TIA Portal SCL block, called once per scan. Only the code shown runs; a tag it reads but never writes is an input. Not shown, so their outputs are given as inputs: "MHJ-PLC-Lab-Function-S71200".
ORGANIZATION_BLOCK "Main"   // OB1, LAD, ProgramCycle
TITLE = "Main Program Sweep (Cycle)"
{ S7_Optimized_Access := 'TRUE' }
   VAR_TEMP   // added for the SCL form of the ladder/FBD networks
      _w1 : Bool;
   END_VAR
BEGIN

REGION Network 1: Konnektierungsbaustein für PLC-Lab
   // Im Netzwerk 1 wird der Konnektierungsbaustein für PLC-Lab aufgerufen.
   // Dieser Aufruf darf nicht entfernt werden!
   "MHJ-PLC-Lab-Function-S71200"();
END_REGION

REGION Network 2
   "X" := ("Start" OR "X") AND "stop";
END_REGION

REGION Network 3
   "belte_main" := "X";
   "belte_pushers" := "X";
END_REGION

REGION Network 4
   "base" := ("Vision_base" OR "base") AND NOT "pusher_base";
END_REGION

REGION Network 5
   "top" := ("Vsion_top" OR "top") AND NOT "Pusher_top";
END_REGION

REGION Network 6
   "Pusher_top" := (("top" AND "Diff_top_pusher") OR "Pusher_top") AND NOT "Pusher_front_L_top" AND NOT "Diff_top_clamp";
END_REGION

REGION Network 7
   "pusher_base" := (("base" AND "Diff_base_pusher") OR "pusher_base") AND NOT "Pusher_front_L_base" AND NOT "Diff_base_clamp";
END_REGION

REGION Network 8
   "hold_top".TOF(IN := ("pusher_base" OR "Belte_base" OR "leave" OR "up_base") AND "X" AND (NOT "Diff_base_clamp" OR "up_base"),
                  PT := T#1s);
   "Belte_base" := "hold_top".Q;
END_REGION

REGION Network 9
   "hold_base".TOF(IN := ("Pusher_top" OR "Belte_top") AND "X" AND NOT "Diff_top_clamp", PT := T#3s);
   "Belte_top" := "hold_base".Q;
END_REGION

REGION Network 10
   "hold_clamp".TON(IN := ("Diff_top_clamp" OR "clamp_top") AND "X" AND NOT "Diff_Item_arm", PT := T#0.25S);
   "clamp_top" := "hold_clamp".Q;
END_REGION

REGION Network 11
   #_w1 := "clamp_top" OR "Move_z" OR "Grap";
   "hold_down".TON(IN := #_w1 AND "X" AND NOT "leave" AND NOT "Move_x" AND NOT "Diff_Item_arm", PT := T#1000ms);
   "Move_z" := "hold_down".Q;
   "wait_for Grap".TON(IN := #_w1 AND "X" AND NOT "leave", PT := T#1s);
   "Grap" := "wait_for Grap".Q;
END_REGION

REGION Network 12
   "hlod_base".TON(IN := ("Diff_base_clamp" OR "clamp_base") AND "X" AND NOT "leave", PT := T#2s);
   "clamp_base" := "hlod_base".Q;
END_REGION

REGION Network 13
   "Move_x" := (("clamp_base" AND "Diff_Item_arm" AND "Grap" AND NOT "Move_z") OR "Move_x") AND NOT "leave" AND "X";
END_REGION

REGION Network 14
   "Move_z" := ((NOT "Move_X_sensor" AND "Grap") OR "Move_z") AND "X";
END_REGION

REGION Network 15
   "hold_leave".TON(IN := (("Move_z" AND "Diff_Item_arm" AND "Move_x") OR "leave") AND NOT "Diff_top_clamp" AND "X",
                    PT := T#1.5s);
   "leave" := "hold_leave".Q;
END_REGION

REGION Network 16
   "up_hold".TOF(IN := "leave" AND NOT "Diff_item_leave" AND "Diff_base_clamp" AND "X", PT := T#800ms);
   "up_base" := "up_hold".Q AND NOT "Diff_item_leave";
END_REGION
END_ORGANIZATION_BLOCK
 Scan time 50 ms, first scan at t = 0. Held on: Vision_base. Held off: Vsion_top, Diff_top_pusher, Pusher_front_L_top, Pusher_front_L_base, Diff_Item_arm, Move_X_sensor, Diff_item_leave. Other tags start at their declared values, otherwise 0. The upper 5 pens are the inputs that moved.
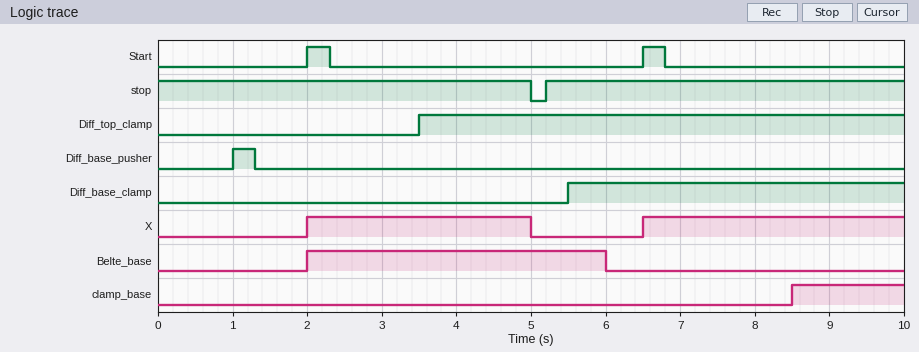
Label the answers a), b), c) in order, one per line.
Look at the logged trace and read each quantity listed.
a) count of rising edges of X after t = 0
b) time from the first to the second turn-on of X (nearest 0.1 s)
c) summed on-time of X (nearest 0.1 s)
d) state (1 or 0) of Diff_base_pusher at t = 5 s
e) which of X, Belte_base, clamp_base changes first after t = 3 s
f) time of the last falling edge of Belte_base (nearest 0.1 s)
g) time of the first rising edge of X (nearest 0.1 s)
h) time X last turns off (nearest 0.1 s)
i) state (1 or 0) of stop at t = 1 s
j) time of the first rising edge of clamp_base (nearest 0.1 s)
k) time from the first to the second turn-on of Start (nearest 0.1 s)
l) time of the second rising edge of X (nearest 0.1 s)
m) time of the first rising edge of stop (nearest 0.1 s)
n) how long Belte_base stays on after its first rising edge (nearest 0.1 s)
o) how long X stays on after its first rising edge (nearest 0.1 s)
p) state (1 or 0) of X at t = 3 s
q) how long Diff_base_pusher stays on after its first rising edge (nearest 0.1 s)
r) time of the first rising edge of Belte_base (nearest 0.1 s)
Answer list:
a) 2
b) 4.5 s
c) 6.5 s
d) 0
e) X
f) 6.0 s
g) 2.0 s
h) 5.0 s
i) 1
j) 8.5 s
k) 4.5 s
l) 6.5 s
m) 5.2 s
n) 4.0 s
o) 3.0 s
p) 1
q) 0.3 s
r) 2.0 s
